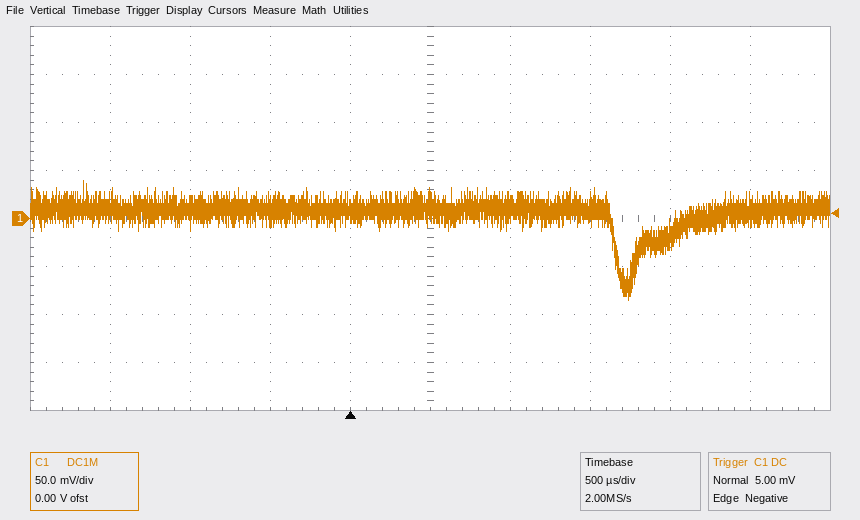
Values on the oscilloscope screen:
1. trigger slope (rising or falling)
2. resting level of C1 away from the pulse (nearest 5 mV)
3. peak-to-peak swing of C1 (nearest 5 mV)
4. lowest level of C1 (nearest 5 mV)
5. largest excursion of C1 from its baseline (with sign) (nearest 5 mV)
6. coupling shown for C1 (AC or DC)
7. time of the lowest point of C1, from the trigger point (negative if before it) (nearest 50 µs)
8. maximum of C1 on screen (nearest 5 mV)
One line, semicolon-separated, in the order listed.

falling; 10 mV; 125 mV; -85 mV; -95 mV; DC; +1.75 ms; 40 mV
